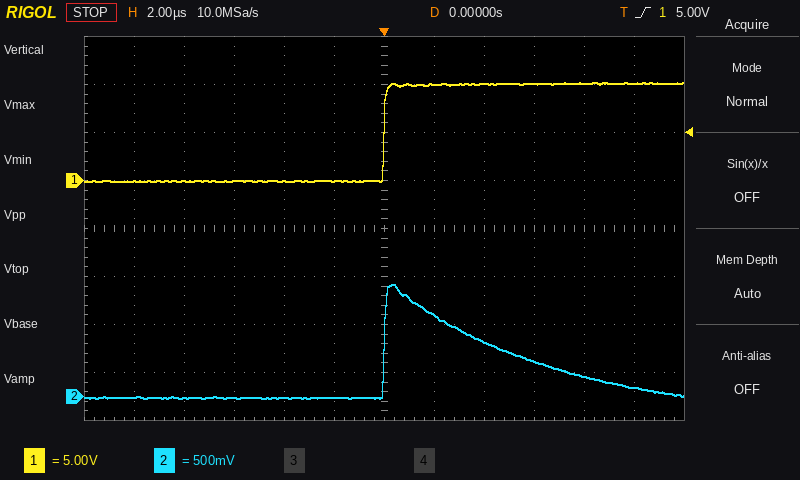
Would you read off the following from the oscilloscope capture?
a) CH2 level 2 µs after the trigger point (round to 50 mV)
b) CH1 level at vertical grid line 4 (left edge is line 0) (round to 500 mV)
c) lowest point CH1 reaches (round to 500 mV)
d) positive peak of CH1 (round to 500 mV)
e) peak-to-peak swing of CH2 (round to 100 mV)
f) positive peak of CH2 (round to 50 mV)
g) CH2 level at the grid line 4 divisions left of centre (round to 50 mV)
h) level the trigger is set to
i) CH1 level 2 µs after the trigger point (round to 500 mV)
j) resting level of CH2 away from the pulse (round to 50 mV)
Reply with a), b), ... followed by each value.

a) 850 mV
b) 0.0 V
c) 0.0 V
d) 10.0 V
e) 1.20 V
f) 1.15 V
g) 0 mV
h) 5.00 V
i) 10.0 V
j) 0 mV
